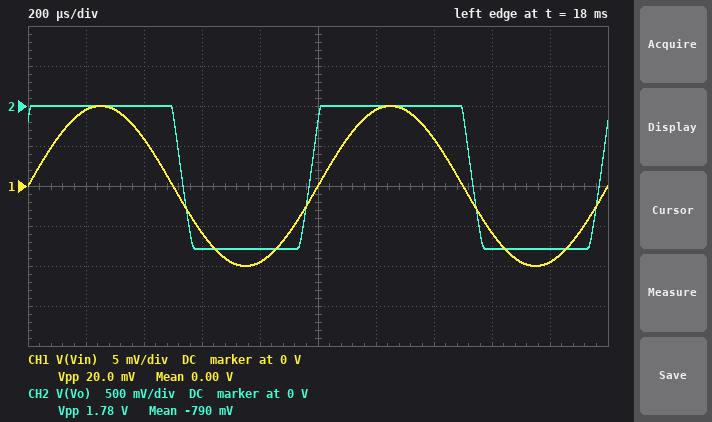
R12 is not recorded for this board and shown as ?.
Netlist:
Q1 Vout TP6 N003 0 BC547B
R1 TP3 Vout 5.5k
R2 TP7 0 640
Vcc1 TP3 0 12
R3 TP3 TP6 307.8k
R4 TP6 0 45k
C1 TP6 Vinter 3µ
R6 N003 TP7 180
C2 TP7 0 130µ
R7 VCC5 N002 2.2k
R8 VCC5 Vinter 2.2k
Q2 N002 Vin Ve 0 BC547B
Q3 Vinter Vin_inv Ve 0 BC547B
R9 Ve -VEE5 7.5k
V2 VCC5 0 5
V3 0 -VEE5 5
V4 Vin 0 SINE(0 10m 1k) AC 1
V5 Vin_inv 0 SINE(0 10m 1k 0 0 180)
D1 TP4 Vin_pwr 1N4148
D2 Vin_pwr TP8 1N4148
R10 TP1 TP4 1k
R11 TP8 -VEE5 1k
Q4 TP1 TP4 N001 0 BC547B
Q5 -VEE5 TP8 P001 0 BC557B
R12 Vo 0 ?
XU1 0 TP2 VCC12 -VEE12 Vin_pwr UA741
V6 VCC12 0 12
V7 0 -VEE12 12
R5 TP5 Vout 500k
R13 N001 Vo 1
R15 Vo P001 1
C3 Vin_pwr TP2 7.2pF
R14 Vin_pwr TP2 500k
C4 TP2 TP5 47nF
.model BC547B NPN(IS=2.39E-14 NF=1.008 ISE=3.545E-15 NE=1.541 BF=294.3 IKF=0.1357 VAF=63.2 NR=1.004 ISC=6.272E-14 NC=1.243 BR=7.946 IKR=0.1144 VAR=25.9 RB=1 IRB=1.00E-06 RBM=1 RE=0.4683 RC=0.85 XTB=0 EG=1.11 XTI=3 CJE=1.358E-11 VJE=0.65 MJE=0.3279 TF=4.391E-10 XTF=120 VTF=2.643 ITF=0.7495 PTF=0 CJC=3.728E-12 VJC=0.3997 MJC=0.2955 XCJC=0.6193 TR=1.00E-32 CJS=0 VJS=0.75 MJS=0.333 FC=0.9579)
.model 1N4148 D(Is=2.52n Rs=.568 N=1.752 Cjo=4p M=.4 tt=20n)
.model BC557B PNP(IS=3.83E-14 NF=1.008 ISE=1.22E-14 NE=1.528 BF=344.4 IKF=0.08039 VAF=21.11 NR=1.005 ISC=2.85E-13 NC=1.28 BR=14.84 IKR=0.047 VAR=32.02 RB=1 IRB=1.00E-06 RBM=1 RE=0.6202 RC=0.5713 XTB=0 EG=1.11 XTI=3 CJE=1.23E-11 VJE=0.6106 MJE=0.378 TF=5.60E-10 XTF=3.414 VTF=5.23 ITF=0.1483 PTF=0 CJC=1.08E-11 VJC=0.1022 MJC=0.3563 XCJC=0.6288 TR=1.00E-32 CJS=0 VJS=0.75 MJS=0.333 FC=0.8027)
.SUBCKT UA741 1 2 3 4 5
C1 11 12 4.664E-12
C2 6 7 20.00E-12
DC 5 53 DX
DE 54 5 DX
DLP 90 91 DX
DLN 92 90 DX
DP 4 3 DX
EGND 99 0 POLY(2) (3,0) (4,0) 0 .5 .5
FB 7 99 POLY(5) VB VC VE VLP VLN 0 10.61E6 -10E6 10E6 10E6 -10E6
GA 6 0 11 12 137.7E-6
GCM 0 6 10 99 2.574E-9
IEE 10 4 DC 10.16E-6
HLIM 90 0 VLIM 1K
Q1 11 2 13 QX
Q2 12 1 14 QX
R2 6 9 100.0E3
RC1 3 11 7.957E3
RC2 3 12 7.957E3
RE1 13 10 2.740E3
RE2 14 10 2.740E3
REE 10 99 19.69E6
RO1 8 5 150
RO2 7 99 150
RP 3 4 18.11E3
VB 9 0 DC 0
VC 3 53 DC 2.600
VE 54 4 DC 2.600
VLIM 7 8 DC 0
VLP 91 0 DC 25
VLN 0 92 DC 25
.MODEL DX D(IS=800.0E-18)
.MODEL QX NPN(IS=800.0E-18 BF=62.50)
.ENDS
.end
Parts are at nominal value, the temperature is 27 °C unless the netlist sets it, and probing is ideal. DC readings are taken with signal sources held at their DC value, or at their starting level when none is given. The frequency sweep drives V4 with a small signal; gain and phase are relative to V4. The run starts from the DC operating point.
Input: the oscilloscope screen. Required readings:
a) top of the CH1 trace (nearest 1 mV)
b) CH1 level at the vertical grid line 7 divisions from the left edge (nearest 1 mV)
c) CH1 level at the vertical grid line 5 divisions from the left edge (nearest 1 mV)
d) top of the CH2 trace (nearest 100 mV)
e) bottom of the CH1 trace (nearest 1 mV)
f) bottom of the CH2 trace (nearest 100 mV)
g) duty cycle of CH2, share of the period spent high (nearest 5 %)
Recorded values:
10 mV
6 mV
0 V
0 V
-10 mV
-1.8 V
55 %
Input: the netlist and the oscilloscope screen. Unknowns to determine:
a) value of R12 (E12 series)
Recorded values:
8.2 Ω
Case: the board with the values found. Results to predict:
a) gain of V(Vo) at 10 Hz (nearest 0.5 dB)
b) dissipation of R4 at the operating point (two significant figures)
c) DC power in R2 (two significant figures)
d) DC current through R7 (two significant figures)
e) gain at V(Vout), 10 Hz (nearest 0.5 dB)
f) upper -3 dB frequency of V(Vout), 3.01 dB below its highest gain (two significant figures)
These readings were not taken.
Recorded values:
29.0 dB
44 µW
570 µW
290 µA
47.0 dB
1.3 MHz
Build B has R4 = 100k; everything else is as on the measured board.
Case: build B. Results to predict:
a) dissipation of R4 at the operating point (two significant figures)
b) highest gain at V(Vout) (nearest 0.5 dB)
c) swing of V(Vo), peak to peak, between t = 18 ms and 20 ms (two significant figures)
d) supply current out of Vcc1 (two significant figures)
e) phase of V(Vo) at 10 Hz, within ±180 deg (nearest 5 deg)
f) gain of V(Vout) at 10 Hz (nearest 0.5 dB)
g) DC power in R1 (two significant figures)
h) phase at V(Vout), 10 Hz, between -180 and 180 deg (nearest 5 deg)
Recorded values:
49 µW
31.0 dB
1.8 V
1.9 mA
100 deg
24.0 dB
19 mW
-115 deg
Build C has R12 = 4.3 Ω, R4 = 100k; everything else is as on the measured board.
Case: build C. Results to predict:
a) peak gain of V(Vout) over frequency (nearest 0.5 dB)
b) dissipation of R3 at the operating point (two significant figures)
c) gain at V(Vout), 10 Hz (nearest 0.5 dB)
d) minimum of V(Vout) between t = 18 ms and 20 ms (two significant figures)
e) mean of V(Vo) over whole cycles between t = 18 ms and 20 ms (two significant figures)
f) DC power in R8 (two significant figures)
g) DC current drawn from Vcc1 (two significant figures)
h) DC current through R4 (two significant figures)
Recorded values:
31.0 dB
310 µW
24.0 dB
1.6 V
-510 mV
190 µW
1.9 mA
22 µA
